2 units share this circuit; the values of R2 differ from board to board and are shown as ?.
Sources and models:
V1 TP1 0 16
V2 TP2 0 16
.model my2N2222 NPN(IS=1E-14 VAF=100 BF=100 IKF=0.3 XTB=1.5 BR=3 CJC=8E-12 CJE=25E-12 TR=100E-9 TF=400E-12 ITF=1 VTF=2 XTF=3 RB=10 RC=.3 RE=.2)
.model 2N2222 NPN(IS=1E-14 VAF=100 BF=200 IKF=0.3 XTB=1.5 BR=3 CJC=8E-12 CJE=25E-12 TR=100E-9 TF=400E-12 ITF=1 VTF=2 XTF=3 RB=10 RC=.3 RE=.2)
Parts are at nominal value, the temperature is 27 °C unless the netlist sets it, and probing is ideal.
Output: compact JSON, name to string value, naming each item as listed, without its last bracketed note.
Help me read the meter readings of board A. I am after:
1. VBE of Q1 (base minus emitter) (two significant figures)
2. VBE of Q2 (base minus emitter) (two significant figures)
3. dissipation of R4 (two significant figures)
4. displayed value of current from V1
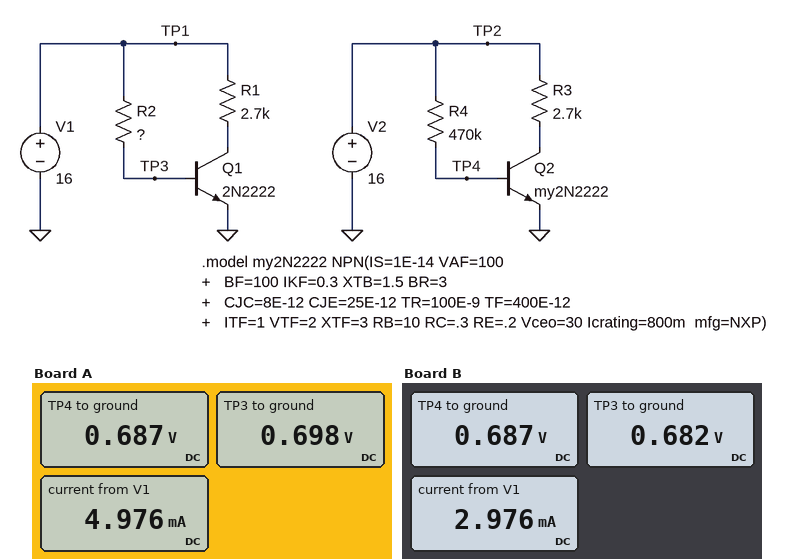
{"VBE of Q1 (base minus emitter)": "700 mV", "VBE of Q2 (base minus emitter)": "690 mV", "dissipation of R4": "500 µW", "displayed value of current from V1": "4.976 mA"}
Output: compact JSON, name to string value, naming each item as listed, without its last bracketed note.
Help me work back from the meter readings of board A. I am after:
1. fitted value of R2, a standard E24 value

{"fitted value of R2, a standard E24 value": "620 kΩ"}
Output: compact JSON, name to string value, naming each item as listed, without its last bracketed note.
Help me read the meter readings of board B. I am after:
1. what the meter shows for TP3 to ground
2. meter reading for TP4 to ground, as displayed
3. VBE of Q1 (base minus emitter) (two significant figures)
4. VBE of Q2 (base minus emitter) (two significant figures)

{"what the meter shows for TP3 to ground": "0.682 V", "meter reading for TP4 to ground, as displayed": "0.687 V", "VBE of Q1 (base minus emitter)": "680 mV", "VBE of Q2 (base minus emitter)": "690 mV"}
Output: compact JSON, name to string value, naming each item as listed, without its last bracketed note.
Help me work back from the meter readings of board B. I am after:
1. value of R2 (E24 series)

{"value of R2": "1.1 MΩ"}
